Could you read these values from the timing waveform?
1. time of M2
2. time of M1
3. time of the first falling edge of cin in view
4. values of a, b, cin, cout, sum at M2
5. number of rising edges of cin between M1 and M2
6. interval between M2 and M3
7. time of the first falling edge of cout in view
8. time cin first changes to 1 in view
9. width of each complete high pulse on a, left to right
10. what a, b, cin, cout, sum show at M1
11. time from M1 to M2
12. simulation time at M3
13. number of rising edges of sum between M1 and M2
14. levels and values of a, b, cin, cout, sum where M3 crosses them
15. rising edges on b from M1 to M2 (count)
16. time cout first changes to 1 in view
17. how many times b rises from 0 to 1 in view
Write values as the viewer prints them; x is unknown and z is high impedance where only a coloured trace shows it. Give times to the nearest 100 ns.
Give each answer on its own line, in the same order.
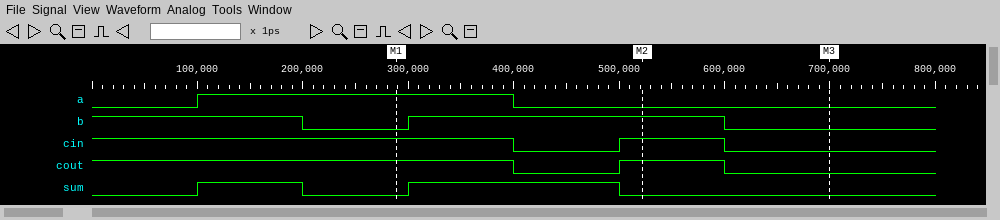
500 ns
300 ns
400 ns
a=0, b=1, cin=1, cout=1, sum=0
1
200 ns
400 ns
500 ns
300 ns
a=1, b=0, cin=1, cout=1, sum=0
200 ns
700 ns
1
a=0, b=0, cin=0, cout=0, sum=0
1
500 ns
1
